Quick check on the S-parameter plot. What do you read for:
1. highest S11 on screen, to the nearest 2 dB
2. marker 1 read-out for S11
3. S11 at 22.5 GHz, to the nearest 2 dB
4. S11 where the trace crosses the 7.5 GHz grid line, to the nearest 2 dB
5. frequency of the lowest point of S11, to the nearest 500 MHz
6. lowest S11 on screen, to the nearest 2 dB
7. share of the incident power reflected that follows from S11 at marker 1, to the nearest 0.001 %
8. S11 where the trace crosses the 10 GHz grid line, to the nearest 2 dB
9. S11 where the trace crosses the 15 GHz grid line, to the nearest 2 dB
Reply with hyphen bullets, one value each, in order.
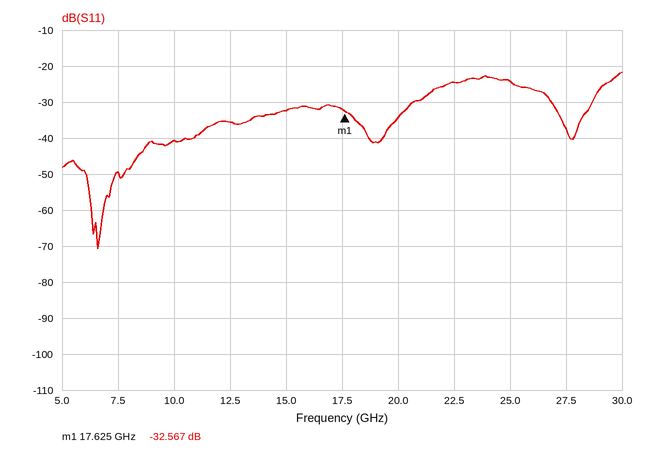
- -22 dB
- -32.567 dB
- -24 dB
- -50 dB
- 6.5 GHz
- -70 dB
- 0.055 %
- -40 dB
- -32 dB
